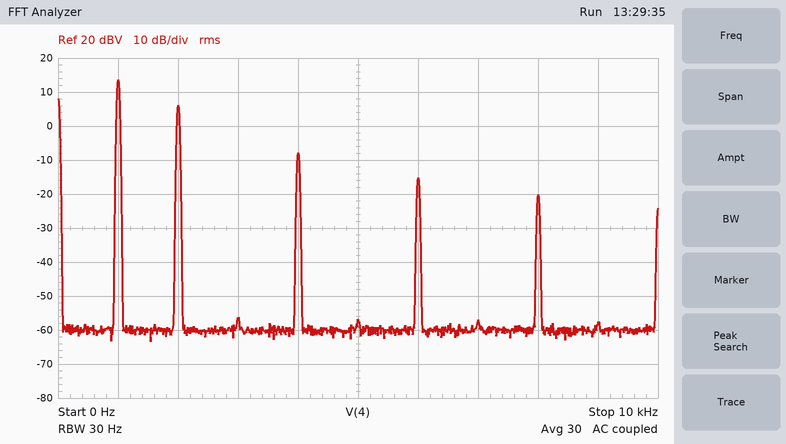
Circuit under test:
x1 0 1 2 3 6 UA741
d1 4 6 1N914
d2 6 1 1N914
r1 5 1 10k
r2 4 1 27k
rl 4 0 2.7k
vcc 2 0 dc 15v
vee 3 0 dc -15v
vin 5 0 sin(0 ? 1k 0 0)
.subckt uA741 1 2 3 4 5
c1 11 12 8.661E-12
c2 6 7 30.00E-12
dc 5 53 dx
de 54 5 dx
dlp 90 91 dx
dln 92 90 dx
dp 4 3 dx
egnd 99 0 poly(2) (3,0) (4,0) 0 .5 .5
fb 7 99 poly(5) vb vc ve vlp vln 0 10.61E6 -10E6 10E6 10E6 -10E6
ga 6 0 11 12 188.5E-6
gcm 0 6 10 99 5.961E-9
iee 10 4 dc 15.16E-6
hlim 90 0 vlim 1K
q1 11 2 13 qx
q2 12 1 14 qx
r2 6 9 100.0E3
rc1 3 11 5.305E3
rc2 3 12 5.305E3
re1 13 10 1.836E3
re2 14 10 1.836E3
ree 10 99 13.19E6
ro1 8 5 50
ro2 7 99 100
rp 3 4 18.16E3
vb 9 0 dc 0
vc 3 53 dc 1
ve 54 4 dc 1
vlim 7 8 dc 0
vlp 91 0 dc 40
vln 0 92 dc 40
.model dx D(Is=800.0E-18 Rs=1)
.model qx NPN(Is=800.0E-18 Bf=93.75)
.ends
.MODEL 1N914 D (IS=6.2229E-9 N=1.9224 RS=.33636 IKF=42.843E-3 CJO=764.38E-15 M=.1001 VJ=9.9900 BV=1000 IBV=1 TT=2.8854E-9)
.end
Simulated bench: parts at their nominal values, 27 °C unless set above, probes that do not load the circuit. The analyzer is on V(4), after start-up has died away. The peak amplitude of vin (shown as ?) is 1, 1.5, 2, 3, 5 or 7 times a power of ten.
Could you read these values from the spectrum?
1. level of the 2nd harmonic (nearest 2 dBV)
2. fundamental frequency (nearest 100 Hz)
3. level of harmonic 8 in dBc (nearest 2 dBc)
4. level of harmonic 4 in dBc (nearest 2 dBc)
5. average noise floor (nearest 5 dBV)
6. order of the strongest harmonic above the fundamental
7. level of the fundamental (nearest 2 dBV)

6 dBV
1.0 kHz
-34 dBc
-22 dBc
-60 dBV
2
14 dBV
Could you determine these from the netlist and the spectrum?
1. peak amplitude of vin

5 V
